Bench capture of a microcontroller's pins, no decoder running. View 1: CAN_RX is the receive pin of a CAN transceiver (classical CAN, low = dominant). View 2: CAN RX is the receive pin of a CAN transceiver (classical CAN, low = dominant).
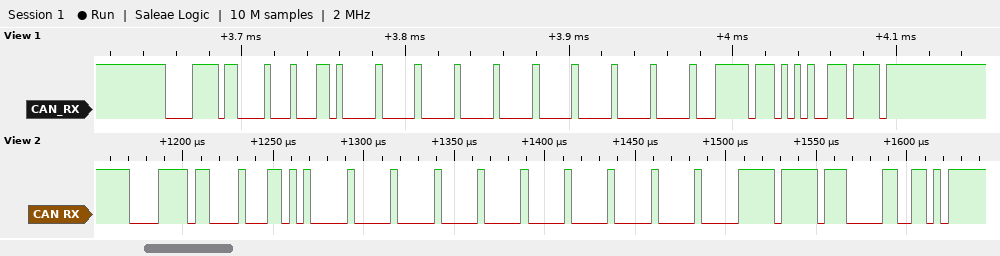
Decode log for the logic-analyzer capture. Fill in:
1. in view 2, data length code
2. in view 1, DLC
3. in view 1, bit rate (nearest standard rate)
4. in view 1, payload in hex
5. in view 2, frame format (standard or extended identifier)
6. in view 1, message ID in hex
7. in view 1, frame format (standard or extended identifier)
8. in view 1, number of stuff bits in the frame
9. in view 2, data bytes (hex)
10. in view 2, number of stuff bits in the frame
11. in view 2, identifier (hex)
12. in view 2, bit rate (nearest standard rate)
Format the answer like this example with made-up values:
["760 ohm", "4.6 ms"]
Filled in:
["8", "8", "250 kbit/s", "8D 00 00 00 00 00 00 FF", "standard", "0x0F6", "standard", "10", "D4 00 00 00 00 00 00 FF", "13", "0x0F6", "250 kbit/s"]
